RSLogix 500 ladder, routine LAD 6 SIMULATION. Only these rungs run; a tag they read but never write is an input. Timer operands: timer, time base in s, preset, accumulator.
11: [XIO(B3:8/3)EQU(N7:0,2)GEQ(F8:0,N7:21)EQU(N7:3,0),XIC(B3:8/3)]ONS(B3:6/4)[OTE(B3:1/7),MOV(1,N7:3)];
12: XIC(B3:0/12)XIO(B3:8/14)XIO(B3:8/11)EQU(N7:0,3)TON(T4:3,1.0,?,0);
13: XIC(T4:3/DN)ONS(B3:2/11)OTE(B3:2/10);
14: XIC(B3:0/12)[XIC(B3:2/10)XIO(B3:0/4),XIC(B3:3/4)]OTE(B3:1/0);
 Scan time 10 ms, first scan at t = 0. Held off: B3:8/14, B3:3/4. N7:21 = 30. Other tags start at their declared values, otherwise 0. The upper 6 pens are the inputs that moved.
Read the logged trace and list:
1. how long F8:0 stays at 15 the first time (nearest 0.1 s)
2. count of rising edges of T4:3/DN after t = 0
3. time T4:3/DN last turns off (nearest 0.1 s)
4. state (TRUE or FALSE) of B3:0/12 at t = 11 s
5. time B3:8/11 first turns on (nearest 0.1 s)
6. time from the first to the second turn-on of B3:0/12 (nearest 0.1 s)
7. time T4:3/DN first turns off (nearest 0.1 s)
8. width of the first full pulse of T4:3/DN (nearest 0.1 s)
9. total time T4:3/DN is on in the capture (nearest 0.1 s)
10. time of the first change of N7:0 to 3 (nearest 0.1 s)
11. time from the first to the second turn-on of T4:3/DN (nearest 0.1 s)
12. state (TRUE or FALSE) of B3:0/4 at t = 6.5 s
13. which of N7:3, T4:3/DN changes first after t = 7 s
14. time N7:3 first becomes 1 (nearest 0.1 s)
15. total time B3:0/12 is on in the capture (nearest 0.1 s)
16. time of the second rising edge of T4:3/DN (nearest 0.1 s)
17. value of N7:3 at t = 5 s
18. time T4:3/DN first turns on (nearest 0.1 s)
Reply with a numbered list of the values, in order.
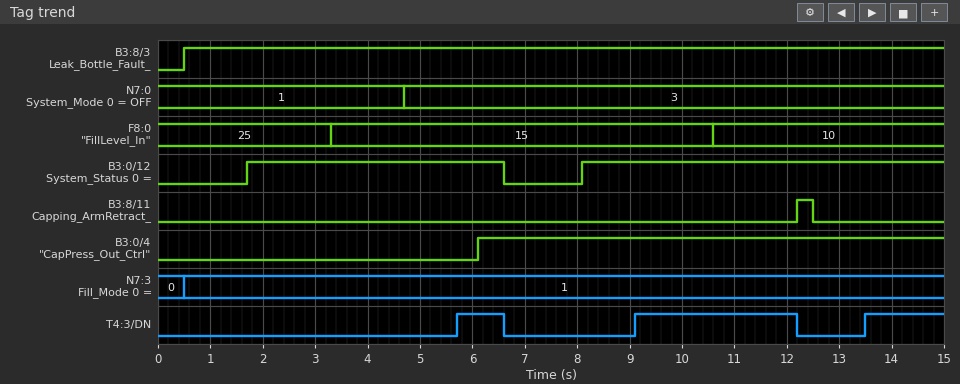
1. 7.3 s
2. 3
3. 12.2 s
4. TRUE
5. 12.2 s
6. 6.4 s
7. 6.6 s
8. 0.9 s
9. 5.5 s
10. 4.7 s
11. 3.4 s
12. TRUE
13. T4:3/DN
14. 0.5 s
15. 11.8 s
16. 9.1 s
17. 1
18. 5.7 s
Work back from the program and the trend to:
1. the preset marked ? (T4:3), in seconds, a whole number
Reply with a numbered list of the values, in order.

1. 1 s
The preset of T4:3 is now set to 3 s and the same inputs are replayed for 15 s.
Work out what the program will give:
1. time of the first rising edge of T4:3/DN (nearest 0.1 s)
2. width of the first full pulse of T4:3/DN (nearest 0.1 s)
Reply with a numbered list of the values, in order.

1. 11.1 s
2. 1.1 s
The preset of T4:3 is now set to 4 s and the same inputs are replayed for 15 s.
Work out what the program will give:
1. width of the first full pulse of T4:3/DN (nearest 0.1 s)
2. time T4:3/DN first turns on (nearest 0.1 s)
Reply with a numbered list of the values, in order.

1. 0.1 s
2. 12.1 s
